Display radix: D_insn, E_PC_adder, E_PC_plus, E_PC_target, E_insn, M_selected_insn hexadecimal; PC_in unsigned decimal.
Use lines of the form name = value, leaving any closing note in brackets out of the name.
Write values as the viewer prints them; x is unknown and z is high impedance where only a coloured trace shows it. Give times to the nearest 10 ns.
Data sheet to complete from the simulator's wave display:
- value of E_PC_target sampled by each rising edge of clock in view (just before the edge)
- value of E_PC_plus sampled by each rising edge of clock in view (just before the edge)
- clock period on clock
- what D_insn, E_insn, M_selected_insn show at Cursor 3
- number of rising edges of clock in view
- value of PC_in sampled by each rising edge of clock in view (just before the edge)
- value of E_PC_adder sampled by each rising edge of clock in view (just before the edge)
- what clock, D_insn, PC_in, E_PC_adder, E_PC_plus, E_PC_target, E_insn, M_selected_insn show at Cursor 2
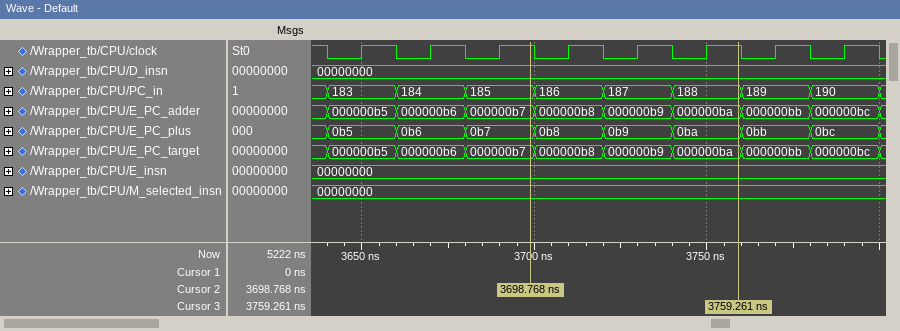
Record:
value of E_PC_target sampled by each rising edge of clock in view = 000000b5, 000000b6, 000000b7, 000000b8, 000000b9, 000000ba, 000000bb, 000000bc
value of E_PC_plus sampled by each rising edge of clock in view = 0b5, 0b6, 0b7, 0b8, 0b9, 0ba, 0bb, 0bc
clock period on clock = 20 ns
what D_insn, E_insn, M_selected_insn show at Cursor 3 = D_insn=00000000, E_insn=00000000, M_selected_insn=00000000
number of rising edges of clock in view = 8
value of PC_in sampled by each rising edge of clock in view = 183, 184, 185, 186, 187, 188, 189, 190
value of E_PC_adder sampled by each rising edge of clock in view = 000000b5, 000000b6, 000000b7, 000000b8, 000000b9, 000000ba, 000000bb, 000000bc
what clock, D_insn, PC_in, E_PC_adder, E_PC_plus, E_PC_target, E_insn, M_selected_insn show at Cursor 2 = clock=1, D_insn=00000000, PC_in=185, E_PC_adder=000000b7, E_PC_plus=0b7, E_PC_target=000000b7, E_insn=00000000, M_selected_insn=00000000
